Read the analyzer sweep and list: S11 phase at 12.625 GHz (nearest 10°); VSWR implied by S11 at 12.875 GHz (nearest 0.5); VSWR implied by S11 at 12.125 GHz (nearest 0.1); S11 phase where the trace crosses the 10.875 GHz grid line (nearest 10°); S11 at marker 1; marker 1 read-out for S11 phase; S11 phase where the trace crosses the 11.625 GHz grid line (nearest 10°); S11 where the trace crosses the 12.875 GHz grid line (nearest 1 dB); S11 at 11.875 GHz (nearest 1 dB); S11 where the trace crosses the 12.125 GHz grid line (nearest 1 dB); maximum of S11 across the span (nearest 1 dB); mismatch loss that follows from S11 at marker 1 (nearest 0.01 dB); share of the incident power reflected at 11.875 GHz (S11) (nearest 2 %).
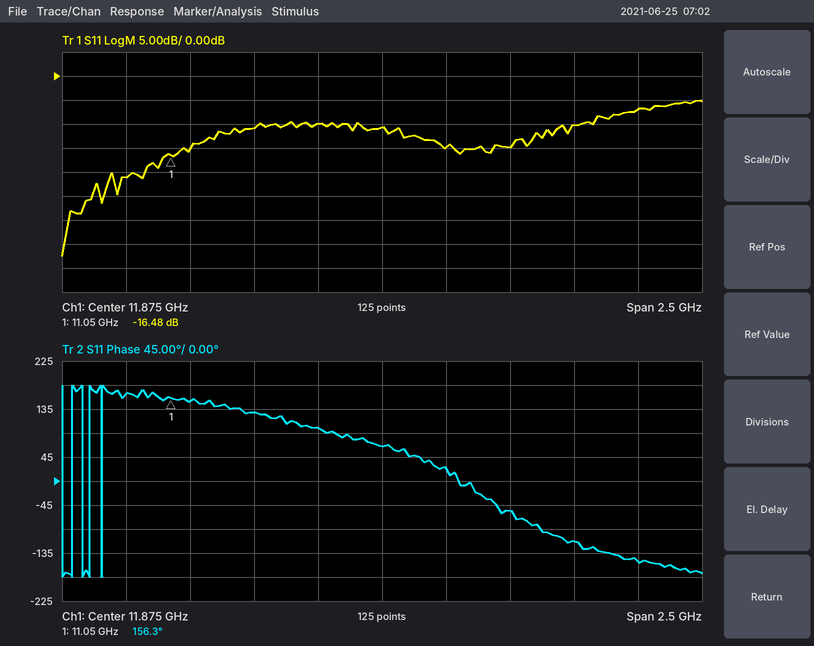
-110°
2.5
1.4
160°
-16.48 dB
156.3°
100°
-7 dB
-11 dB
-15 dB
-5 dB
0.10 dB
8 %
